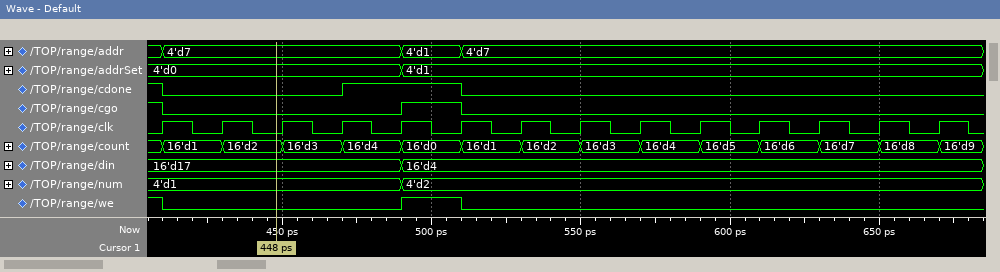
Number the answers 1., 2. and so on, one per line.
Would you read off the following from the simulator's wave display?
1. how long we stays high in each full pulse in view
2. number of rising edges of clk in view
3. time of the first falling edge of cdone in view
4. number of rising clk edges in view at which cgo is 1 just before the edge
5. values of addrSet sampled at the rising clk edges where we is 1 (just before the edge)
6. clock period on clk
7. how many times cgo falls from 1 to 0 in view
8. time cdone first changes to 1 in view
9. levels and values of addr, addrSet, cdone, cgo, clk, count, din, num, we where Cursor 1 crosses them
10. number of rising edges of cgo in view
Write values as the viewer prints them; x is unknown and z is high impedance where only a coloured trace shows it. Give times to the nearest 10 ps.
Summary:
1. 20 ps
2. 14
3. 410 ps
4. 2
5. 4'd0, 4'd1
6. 20 ps
7. 2
8. 470 ps
9. addr=4'd7, addrSet=4'd0, cdone=0, cgo=0, clk=0, count=16'd2, din=16'd17, num=4'd1, we=0
10. 1
